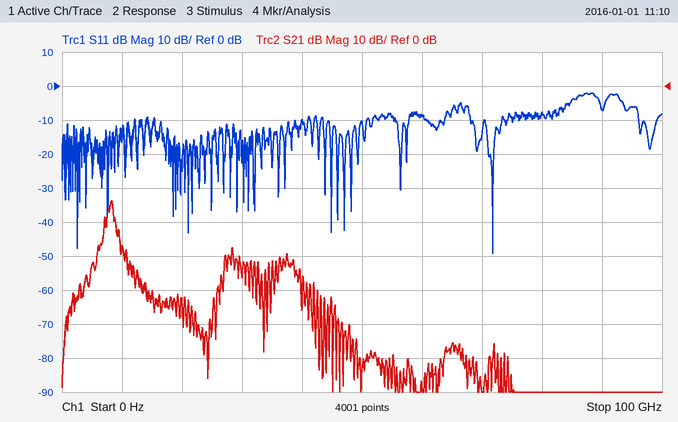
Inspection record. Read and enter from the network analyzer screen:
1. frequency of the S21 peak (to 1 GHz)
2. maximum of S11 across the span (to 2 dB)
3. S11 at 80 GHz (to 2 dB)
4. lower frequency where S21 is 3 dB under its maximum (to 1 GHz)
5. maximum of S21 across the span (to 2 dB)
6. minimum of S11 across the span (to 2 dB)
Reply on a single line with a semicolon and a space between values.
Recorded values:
8 GHz; -2 dB; -8 dB; 8 GHz; -34 dB; -50 dB
